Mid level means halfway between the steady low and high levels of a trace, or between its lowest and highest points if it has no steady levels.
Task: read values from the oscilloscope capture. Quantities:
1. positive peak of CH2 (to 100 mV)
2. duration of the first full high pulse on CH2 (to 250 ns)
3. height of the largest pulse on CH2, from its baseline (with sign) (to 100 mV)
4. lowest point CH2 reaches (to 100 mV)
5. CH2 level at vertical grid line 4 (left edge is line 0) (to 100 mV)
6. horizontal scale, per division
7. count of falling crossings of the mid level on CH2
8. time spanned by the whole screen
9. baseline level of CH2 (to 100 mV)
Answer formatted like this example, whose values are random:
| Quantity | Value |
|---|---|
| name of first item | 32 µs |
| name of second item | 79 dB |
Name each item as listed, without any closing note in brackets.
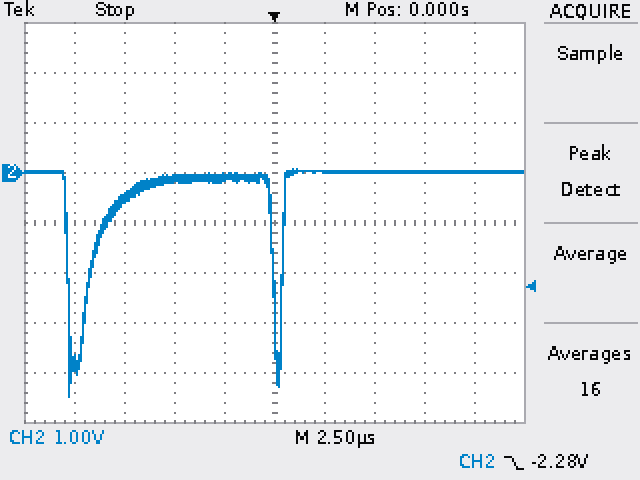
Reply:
| Quantity | Value |
|---|---|
| positive peak of CH2 | 100 mV |
| duration of the first full high pulse on CH2 | 9.25 µs |
| height of the largest pulse on CH2, from its baseline (with sign) | -4.5 V |
| lowest point CH2 reaches | -4.5 V |
| CH2 level at vertical grid line 4 (left edge is line 0) | -100 mV |
| horizontal scale, per division | 2.5 µs |
| count of falling crossings of the mid level on CH2 | 2 |
| time spanned by the whole screen | 25 µs |
| baseline level of CH2 | 0.0 V |
